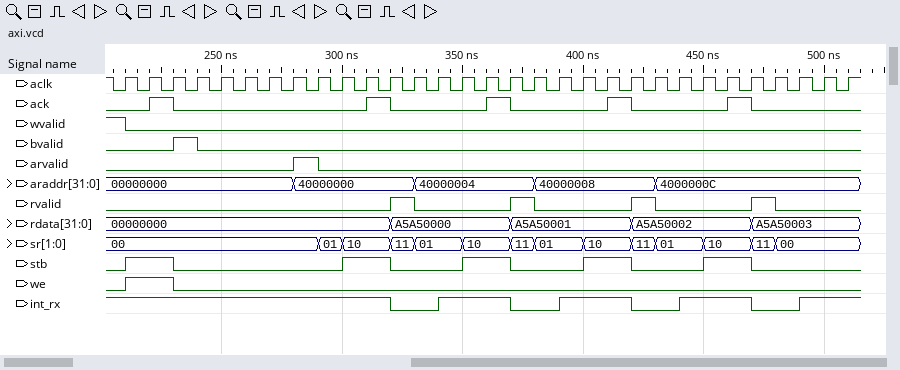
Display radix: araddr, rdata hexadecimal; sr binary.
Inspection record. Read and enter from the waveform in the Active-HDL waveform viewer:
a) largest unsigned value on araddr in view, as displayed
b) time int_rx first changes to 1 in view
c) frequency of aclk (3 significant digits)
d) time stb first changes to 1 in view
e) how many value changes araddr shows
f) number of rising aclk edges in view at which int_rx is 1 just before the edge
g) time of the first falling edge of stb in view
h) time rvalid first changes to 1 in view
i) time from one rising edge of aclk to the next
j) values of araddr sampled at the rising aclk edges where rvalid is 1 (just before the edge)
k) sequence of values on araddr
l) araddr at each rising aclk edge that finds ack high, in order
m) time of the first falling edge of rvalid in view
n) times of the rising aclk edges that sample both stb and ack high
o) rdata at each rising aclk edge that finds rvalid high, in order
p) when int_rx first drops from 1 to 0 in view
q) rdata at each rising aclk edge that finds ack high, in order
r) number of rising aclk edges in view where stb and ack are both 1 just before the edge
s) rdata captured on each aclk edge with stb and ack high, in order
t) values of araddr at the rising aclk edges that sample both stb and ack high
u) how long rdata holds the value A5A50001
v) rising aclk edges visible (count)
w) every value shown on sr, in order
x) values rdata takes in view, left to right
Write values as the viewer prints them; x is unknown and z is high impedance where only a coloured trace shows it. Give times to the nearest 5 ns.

4000000C
340 ns
100 MHz
210 ns
4
23
230 ns
320 ns
10 ns
40000000, 40000004, 40000008, 4000000C
00000000, 40000000, 40000004, 40000008, 4000000C
00000000, 40000000, 40000004, 40000008, 4000000C
330 ns
230 ns, 320 ns, 370 ns, 420 ns, 470 ns
A5A50000, A5A50001, A5A50002, A5A50003
320 ns
00000000, 00000000, A5A50000, A5A50001, A5A50002
5
00000000, 00000000, A5A50000, A5A50001, A5A50002
00000000, 40000000, 40000004, 40000008, 4000000C
50 ns
31
00, 01, 10, 11, 01, 10, 11, 01, 10, 11, 01, 10, 11, 00
00000000, A5A50000, A5A50001, A5A50002, A5A50003
